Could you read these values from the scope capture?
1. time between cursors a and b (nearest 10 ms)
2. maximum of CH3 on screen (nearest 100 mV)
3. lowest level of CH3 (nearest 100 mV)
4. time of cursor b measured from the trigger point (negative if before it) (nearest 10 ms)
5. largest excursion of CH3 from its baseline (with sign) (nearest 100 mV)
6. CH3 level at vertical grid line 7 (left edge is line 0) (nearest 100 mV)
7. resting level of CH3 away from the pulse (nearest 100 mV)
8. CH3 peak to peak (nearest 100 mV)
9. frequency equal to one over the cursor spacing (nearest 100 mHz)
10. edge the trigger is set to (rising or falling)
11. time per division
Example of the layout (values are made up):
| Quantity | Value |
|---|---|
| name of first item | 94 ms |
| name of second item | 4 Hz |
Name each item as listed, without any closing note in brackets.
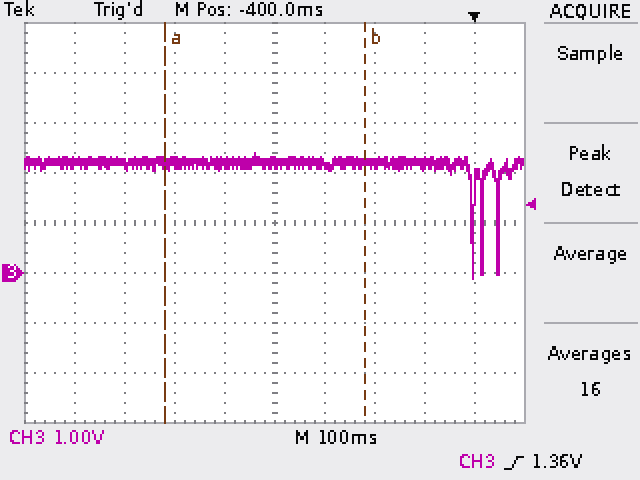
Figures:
| Quantity | Value |
|---|---|
| time between cursors a and b | 400 ms |
| maximum of CH3 on screen | 2.4 V |
| lowest level of CH3 | -100 mV |
| time of cursor b measured from the trigger point (negative if before it) | -220 ms |
| largest excursion of CH3 from its baseline (with sign) | -2.3 V |
| CH3 level at vertical grid line 7 (left edge is line 0) | 2.2 V |
| resting level of CH3 away from the pulse | 2.2 V |
| CH3 peak to peak | 2.5 V |
| frequency equal to one over the cursor spacing | 2.5 Hz |
| edge the trigger is set to | rising |
| time per division | 100 ms |
